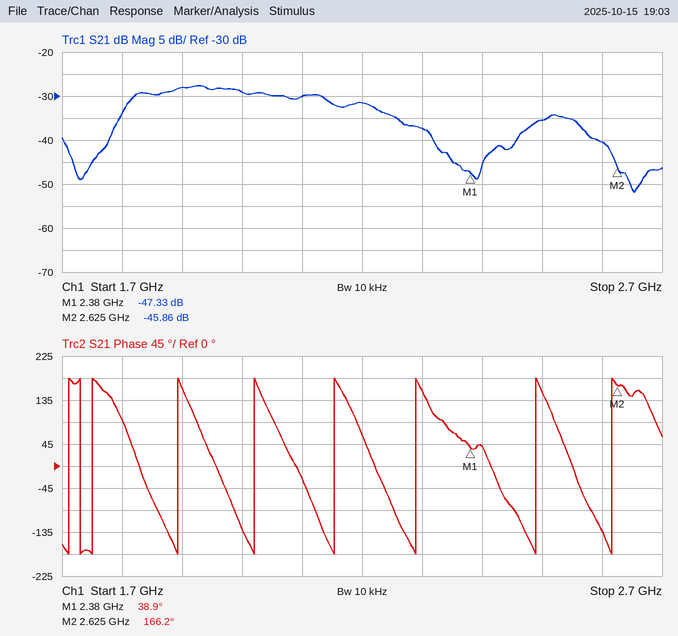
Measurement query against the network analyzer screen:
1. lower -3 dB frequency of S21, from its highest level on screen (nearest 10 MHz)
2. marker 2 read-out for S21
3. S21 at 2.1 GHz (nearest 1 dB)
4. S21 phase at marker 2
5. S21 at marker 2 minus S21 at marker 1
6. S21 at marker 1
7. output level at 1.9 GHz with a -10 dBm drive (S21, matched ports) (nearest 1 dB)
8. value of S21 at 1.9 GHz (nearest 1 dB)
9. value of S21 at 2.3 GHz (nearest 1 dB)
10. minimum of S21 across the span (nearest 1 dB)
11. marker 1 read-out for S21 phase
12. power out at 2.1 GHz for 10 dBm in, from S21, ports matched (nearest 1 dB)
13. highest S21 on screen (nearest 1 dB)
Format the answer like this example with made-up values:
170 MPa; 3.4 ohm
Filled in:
1.82 GHz; -45.86 dB; -30 dB; 166.2°; 1.47 dB; -47.33 dB; -38 dBm; -28 dB; -37 dB; -52 dB; 38.9°; -20 dBm; -28 dB
